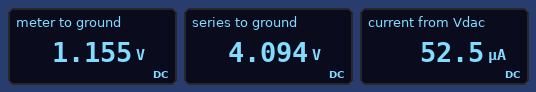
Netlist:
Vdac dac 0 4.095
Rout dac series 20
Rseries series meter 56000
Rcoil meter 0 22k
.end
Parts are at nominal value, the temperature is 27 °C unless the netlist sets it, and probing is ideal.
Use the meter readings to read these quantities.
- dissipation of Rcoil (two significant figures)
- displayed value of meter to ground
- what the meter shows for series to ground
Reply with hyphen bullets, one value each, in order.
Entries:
- 61 µW
- 1.155 V
- 4.094 V
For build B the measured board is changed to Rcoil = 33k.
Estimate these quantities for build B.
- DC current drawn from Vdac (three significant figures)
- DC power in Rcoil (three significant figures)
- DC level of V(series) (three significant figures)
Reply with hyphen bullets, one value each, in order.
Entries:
- 46.0 µA
- 69.8 µW
- 4.09 V
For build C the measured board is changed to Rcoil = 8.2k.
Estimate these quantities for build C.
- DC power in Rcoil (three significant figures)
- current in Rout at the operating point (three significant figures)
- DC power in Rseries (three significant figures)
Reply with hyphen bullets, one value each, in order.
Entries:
- 33.3 µW
- 63.8 µA
- 228 µW
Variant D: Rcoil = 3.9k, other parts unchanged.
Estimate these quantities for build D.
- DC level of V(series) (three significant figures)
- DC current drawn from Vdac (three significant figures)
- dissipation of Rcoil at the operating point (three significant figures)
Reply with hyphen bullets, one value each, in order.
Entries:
- 4.09 V
- 68.3 µA
- 18.2 µW
